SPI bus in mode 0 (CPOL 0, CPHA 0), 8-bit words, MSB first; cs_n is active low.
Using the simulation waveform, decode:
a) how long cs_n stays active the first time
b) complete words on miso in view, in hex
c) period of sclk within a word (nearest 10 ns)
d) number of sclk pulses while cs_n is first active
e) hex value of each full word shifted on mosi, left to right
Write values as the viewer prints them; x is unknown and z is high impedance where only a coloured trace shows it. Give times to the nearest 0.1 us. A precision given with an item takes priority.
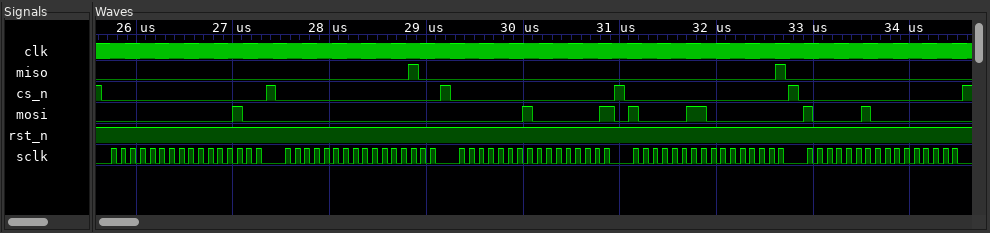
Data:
1.7 us
00, 00, 00, 04, 00, 00, 00, 01, 00, 00
100 ns
16
00, 04, 00, 00, 01, 01, 83, 00, 82, 00
